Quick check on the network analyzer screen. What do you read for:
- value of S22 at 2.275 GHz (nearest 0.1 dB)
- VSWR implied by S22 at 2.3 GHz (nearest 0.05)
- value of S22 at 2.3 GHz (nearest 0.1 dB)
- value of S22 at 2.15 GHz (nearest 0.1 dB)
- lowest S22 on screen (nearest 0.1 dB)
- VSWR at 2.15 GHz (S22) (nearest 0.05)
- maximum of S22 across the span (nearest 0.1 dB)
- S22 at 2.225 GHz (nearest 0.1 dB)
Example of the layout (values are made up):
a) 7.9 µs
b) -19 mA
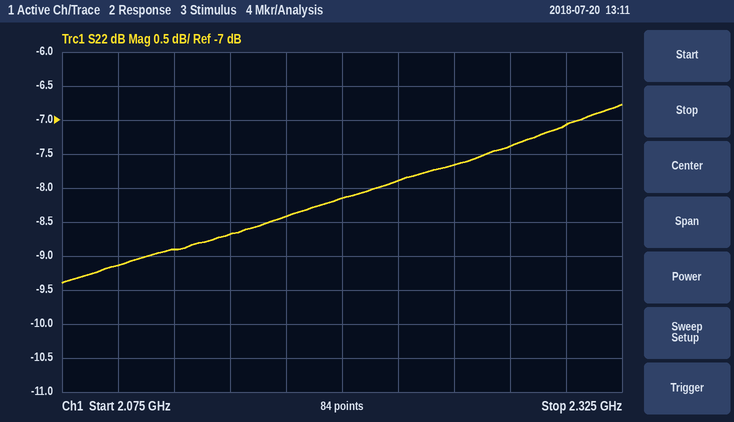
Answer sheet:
a) -7.4 dB
b) 2.60
c) -7.1 dB
d) -8.7 dB
e) -9.4 dB
f) 2.15
g) -6.8 dB
h) -7.9 dB
